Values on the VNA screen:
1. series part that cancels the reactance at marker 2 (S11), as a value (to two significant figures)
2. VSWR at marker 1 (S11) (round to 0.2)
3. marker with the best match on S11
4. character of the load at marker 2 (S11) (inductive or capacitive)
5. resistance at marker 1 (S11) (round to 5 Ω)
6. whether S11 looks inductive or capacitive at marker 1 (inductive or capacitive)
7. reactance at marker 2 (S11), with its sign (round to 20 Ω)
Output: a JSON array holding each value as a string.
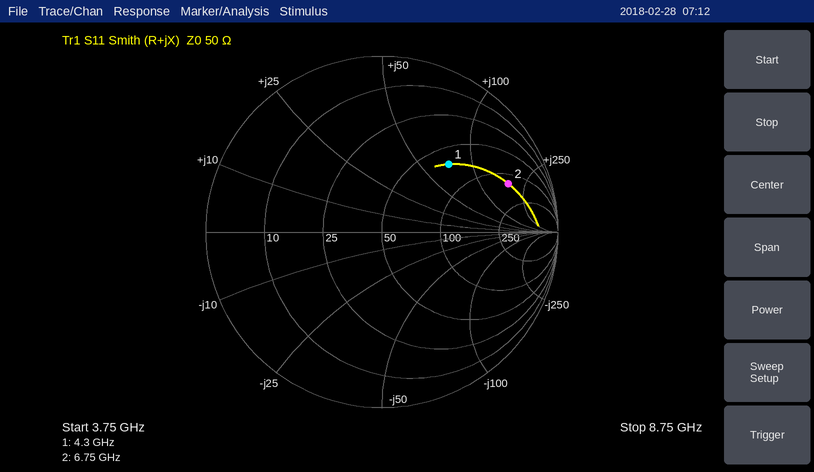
["130 fF", "3.4", "marker 1", "inductive", "65 Ω", "inductive", "+180 Ω"]
